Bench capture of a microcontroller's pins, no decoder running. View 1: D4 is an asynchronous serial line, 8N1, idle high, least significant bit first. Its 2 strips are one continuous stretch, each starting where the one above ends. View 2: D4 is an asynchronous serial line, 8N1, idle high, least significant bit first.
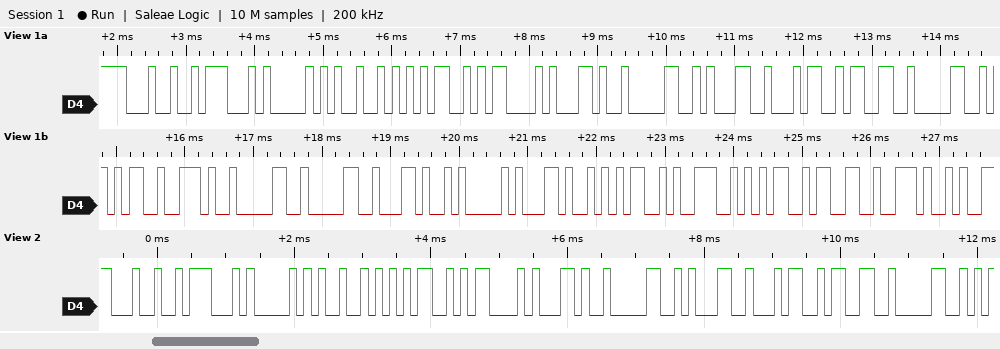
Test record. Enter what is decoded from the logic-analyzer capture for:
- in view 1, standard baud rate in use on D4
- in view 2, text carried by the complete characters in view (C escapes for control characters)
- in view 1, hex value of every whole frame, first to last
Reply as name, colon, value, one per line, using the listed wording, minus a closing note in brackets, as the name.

in view 1, standard baud rate in use on D4: 9600 baud
in view 2, text carried by the complete characters in view: "$GPRMC,01430"
in view 1, hex value of every whole frame, first to last: 0x24 0x47 0x50 0x52 0x4D 0x43 0x2C 0x30 0x31 0x34 0x33 0x30 0x35 0x2E 0x30 0x30 0x2C 0x41 0x2C 0x35 0x39 0x35 0x33 0x2E
